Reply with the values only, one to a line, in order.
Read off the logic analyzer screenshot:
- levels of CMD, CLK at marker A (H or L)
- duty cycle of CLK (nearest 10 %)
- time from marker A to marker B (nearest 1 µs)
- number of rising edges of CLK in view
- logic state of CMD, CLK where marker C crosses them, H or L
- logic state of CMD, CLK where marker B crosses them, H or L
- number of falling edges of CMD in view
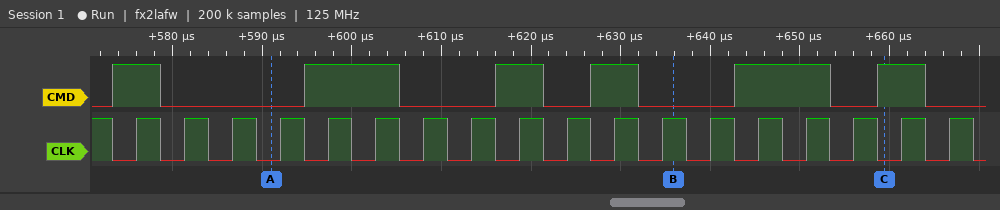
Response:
CMD=L, CLK=L
50 %
45 µs
18
CMD=H, CLK=L
CMD=L, CLK=H
6
